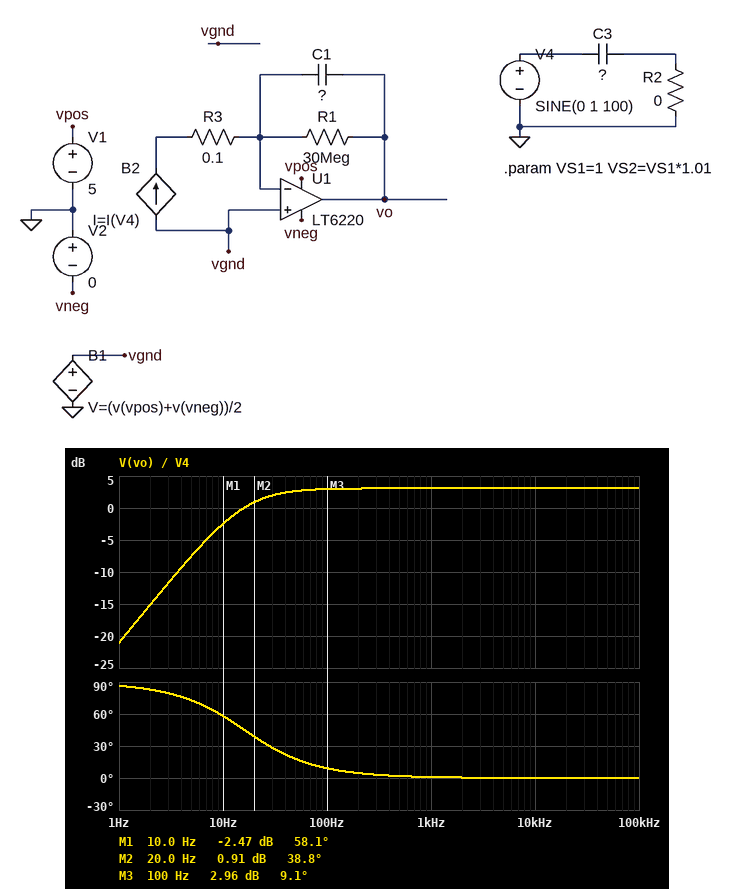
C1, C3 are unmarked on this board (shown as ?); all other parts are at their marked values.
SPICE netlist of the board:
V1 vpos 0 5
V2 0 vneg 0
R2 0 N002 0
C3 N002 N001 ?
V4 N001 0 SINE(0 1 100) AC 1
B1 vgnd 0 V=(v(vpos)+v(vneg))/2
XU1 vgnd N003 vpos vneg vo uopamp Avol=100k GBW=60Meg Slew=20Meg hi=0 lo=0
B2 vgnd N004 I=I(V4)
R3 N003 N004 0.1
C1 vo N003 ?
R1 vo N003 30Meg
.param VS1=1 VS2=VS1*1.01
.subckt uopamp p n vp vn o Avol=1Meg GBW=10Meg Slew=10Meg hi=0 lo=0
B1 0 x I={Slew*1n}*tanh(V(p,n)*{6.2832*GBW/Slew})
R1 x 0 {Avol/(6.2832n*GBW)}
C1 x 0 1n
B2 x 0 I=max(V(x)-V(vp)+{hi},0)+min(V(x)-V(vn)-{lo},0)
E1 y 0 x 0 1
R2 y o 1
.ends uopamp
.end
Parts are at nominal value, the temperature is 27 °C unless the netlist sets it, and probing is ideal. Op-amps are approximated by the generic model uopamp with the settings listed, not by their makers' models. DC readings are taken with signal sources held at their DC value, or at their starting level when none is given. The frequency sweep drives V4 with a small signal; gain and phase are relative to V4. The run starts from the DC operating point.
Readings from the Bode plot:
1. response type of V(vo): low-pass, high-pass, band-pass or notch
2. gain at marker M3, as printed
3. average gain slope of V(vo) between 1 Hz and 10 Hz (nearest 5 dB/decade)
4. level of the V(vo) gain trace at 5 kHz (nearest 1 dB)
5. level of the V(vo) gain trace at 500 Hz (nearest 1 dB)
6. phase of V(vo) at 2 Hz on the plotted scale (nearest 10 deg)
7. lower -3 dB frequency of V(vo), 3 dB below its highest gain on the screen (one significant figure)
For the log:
high-pass
2.96 dB
20 dB/decade
3 dB
3 dB
80 deg
20 Hz
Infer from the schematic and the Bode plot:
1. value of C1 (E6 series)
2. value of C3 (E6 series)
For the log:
330 pF
470 pF
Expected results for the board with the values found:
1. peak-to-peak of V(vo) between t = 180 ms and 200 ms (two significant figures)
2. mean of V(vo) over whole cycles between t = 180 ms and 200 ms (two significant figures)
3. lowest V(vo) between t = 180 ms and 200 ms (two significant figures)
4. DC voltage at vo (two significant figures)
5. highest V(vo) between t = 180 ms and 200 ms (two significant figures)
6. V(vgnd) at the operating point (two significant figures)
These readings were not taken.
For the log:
2.8 V
2.5 V
1.1 V
2.5 V
3.9 V
2.5 V
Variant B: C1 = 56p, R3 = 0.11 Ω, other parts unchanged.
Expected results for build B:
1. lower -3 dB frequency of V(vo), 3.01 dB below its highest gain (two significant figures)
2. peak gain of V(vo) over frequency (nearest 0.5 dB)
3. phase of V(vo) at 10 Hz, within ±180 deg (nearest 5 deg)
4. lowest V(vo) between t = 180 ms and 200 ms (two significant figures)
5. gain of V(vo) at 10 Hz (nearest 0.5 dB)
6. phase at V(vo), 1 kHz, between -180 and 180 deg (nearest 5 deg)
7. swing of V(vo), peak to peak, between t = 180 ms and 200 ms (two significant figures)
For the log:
95 Hz
18.5 dB
85 deg
-20 mV
-1.0 dB
5 deg
5.0 V
